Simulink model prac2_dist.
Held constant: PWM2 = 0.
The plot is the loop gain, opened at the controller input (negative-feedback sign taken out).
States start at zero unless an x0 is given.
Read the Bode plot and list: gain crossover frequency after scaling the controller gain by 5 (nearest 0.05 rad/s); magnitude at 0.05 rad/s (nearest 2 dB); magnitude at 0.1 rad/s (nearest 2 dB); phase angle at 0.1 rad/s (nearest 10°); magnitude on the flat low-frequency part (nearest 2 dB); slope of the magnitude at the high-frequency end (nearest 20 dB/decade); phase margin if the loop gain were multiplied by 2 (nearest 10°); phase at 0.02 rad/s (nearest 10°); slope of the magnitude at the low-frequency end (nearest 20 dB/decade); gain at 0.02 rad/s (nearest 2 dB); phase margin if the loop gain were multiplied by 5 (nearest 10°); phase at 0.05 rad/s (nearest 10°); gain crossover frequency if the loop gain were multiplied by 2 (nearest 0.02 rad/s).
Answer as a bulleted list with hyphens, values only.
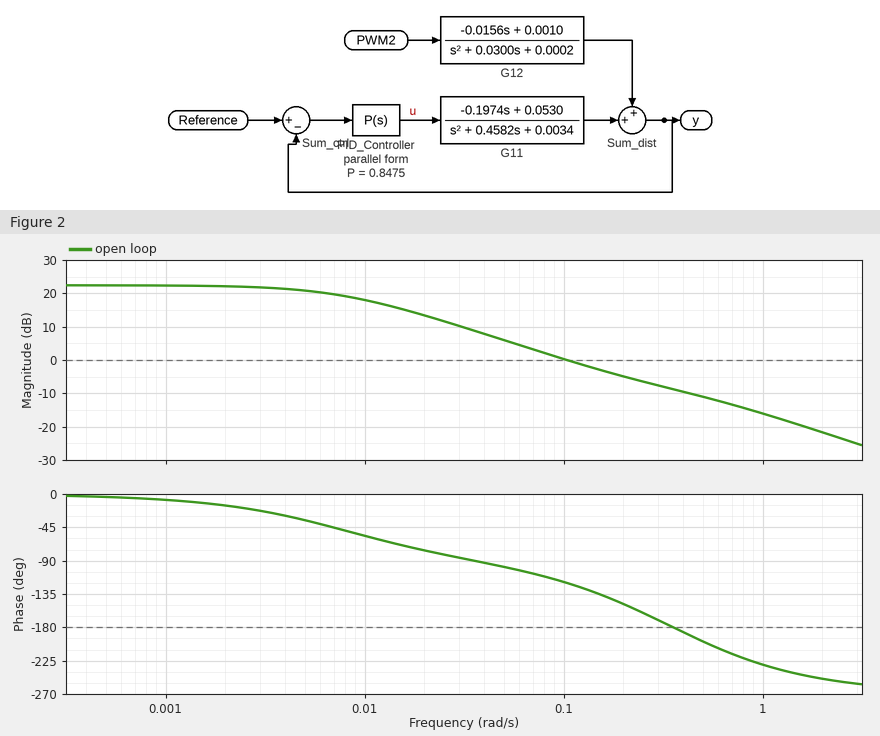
- 0.75 rad/s
- 6 dB
- 0 dB
- -120°
- 22 dB
- -20 dB/decade
- 20°
- -80°
- 0 dB/decade
- 14 dB
- -40°
- -100°
- 0.24 rad/s
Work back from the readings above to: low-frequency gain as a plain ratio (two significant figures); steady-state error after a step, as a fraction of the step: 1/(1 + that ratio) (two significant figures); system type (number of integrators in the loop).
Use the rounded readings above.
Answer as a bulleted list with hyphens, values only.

- 13
- 0.071
- 0
